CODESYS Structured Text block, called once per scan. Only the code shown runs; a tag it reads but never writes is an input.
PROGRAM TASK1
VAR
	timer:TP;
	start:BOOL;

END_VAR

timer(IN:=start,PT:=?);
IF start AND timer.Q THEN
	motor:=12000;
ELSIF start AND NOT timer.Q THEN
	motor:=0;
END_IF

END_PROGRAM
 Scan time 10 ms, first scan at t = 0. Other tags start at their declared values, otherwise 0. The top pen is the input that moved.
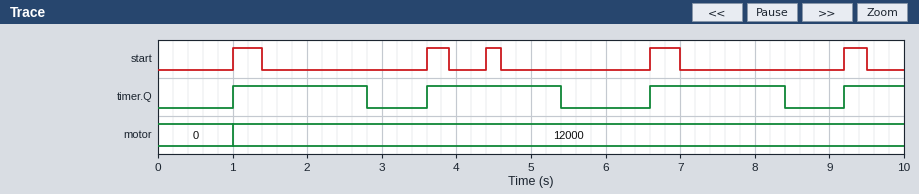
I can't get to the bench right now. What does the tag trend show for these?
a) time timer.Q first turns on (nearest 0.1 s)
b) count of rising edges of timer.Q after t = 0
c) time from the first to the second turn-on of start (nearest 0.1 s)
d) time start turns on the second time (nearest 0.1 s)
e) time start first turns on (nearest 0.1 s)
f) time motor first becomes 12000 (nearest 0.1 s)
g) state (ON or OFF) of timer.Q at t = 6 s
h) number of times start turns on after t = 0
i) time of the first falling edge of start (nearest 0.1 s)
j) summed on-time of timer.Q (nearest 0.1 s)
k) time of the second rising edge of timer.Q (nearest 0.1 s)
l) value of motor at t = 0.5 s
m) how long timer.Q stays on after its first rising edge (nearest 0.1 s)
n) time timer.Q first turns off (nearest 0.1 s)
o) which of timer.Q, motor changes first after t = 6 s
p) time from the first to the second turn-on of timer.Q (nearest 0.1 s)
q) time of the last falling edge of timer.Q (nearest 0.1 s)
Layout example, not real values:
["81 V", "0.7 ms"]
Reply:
["1.0 s", "4", "2.6 s", "3.6 s", "1.0 s", "1.0 s", "OFF", "5", "1.4 s", "6.2 s", "3.6 s", "0", "1.8 s", "2.8 s", "timer.Q", "2.6 s", "8.4 s"]
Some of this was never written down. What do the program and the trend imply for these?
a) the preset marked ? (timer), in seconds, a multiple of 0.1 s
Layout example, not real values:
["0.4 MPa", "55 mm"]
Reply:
["1.8 s"]
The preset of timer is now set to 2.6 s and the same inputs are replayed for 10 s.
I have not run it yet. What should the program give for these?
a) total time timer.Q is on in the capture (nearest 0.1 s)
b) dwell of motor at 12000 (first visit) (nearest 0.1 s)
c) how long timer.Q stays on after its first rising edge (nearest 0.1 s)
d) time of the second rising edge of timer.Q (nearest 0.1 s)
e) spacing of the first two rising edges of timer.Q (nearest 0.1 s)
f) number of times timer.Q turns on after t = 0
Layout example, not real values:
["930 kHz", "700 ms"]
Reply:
["6.0 s", "2.6 s", "2.6 s", "4.4 s", "3.4 s", "3"]
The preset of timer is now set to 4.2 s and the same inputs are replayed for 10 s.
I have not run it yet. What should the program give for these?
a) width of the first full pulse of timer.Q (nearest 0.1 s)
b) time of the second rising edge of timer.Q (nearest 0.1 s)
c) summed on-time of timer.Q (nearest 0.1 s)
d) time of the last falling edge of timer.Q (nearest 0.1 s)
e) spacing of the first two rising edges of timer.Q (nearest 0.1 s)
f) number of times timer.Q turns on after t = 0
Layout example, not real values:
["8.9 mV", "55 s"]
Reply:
["4.2 s", "6.6 s", "7.6 s", "5.2 s", "5.6 s", "2"]
